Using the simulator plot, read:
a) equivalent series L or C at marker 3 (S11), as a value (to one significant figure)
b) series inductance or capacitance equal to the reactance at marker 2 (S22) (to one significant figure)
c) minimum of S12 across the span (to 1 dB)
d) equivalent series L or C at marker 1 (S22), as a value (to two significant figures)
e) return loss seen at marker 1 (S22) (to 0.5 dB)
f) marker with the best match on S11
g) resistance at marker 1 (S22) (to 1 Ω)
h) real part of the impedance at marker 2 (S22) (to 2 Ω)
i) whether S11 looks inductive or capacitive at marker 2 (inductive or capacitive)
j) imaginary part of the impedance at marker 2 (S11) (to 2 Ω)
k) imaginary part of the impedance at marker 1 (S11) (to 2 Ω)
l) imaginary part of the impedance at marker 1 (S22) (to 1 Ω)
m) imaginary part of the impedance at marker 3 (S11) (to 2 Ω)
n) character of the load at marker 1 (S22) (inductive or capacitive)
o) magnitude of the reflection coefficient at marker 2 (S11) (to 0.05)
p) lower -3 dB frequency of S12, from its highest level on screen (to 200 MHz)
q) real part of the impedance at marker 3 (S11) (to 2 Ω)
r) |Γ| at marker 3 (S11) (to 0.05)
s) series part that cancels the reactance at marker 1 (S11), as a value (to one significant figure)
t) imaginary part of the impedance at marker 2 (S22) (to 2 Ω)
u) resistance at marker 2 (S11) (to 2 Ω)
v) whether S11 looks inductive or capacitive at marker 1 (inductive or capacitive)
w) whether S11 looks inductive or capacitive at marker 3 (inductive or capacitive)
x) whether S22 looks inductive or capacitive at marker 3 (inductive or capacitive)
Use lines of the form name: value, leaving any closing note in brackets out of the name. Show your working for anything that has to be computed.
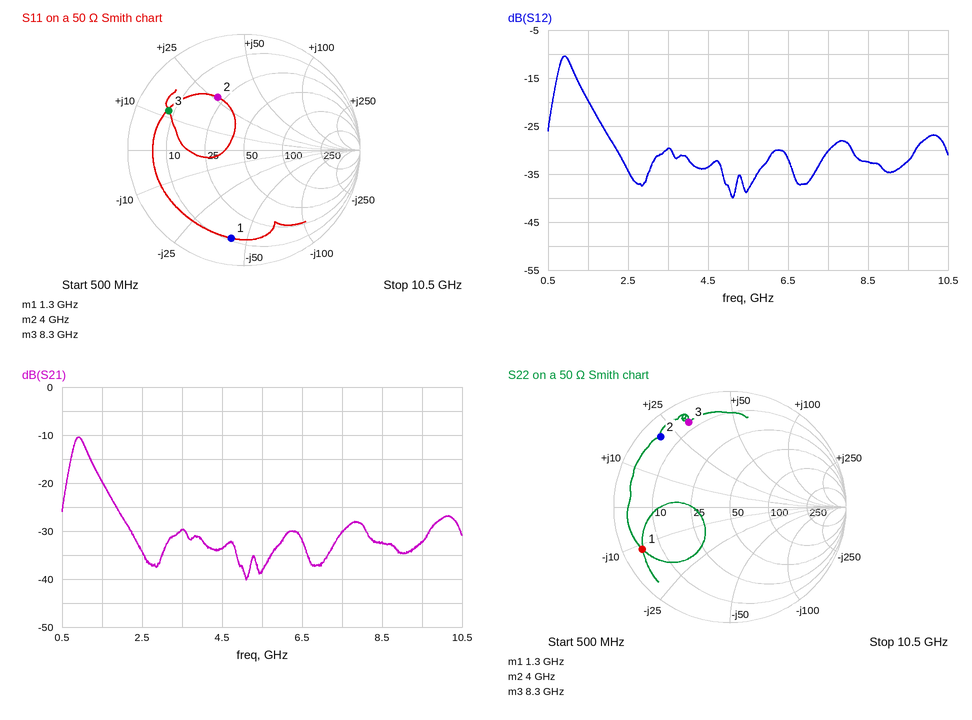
equivalent series L or C at marker 3 (S11), as a value: L = 12 Ω/(2π × 8.3 GHz) ≈ 230 pH, so 200 pH to one significant figure
series inductance or capacitance equal to the reactance at marker 2 (S22): L = 20 Ω/(2π × 4 GHz) ≈ 796 pH, so 800 pH to one significant figure
minimum of S12 across the span: -40 dB
equivalent series L or C at marker 1 (S22), as a value: C = 1/(2π × 1.3 GHz × 11 Ω) ≈ 11 pF
return loss seen at marker 1 (S22): 1.5 dB
marker with the best match on S11: marker 2
resistance at marker 1 (S22): 5 Ω
real part of the impedance at marker 2 (S22): 4 Ω
whether S11 looks inductive or capacitive at marker 2: inductive
imaginary part of the impedance at marker 2 (S11): +26 Ω
imaginary part of the impedance at marker 1 (S11): -42 Ω
imaginary part of the impedance at marker 1 (S22): -11 Ω
imaginary part of the impedance at marker 3 (S11): +12 Ω
character of the load at marker 1 (S22): capacitive
magnitude of the reflection coefficient at marker 2 (S11): 0.50
lower -3 dB frequency of S12, from its highest level on screen: 800 MHz
real part of the impedance at marker 3 (S11): 8 Ω
|Γ| at marker 3 (S11): 0.75
series part that cancels the reactance at marker 1 (S11), as a value: L = 42 Ω/(2π × 1.3 GHz) ≈ 5 nH
imaginary part of the impedance at marker 2 (S22): +20 Ω
resistance at marker 2 (S11): 22 Ω
whether S11 looks inductive or capacitive at marker 1: capacitive
whether S11 looks inductive or capacitive at marker 3: inductive
whether S22 looks inductive or capacitive at marker 3: inductive
